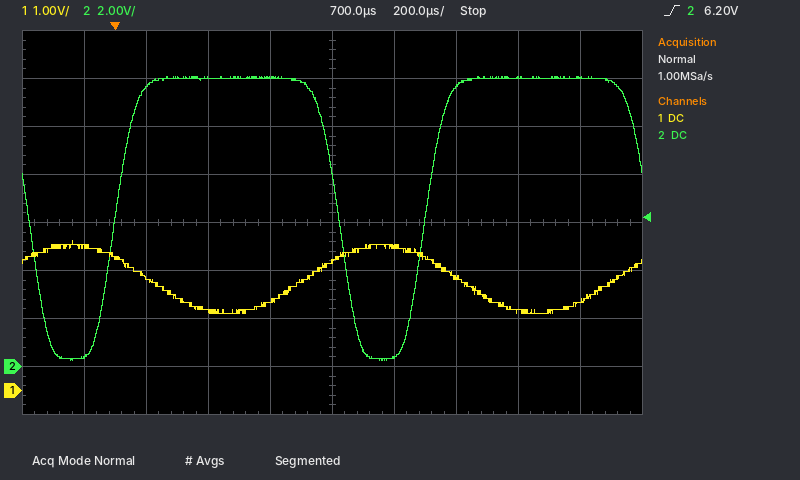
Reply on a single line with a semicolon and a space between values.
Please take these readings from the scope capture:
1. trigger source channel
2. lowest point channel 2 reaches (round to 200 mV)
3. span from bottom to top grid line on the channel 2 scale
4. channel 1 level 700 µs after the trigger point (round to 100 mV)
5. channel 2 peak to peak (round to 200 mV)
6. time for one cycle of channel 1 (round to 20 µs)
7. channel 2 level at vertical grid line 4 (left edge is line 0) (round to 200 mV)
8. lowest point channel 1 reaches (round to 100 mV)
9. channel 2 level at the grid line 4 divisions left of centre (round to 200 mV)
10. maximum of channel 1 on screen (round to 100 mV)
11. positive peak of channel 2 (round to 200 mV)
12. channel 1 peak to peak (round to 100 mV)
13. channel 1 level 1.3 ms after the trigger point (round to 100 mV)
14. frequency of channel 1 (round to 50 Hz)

channel 2; 200 mV; 16 V; 2.7 V; 11.8 V; 1.00 ms; 12.0 V; 1.6 V; 400 mV; 3.1 V; 12.0 V; 1.5 V; 1.6 V; 1.00 kHz
